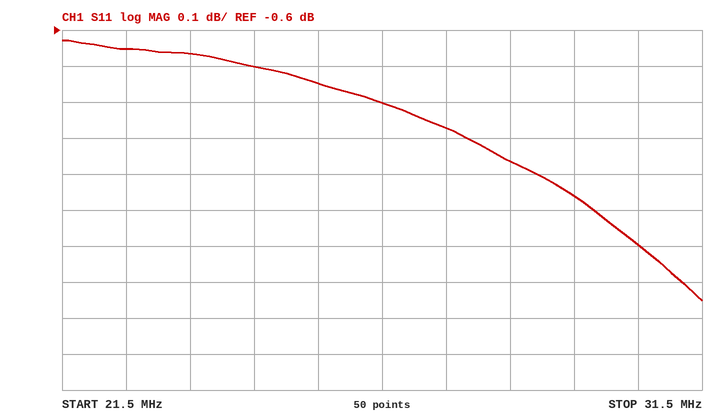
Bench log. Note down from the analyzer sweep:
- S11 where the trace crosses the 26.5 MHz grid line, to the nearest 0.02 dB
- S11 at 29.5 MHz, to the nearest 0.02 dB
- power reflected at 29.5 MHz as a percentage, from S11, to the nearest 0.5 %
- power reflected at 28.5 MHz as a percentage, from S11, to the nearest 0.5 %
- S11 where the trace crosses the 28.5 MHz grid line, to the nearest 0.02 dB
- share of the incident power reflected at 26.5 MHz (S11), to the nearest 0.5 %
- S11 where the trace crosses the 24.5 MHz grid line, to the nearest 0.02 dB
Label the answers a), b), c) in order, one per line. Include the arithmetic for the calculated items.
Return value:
a) -0.80 dB
b) -1.06 dB
c) 10^(-1.06/10) ≈ 78.3 %, so 78.5 % to the nearest 0.5 %
d) 10^(-0.96/10) ≈ 80.2 %, so 80.0 % to the nearest 0.5 %
e) -0.96 dB
f) 10^(-0.8/10) ≈ 83.2 %, so 83.0 % to the nearest 0.5 %
g) -0.70 dB
